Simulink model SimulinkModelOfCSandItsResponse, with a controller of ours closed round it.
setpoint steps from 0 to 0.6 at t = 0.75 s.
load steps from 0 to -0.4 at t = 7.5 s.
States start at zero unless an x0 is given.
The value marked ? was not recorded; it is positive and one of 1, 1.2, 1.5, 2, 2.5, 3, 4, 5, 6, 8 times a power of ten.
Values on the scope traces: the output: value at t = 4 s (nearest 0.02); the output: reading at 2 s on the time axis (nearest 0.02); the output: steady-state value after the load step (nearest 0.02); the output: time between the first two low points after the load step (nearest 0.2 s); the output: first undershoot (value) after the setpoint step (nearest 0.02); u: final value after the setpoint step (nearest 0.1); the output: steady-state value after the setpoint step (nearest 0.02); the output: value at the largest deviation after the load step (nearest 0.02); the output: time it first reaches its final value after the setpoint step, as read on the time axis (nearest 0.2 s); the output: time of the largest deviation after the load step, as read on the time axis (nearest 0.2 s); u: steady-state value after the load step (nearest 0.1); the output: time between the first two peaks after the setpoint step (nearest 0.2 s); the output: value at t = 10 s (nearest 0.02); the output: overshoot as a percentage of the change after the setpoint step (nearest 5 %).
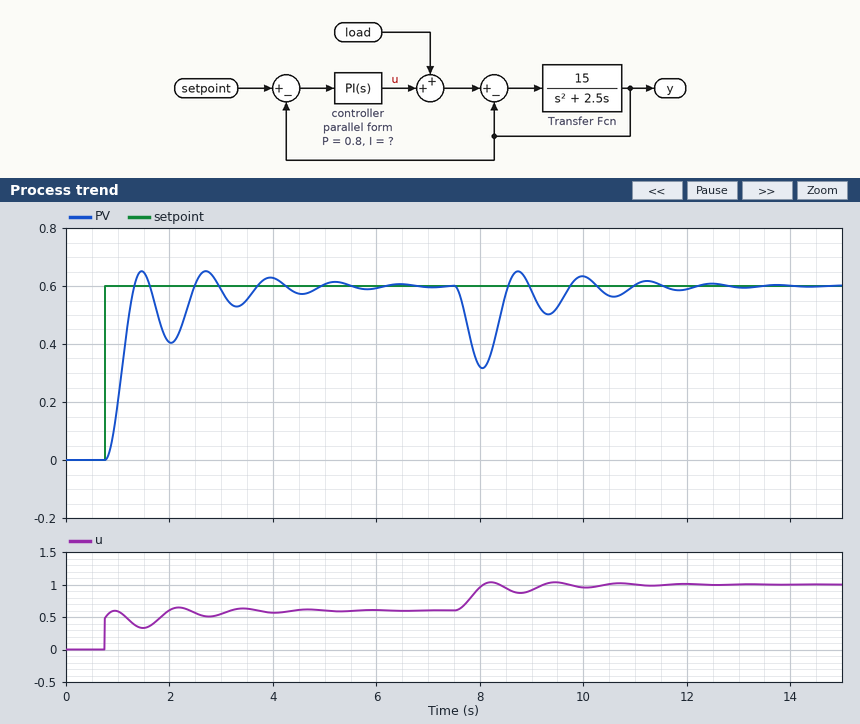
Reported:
0.62
0.40
0.60
1.2 s
0.40
0.6
0.60
0.32
1.4 s
8.0 s
1.0
1.2 s
0.64
10 %
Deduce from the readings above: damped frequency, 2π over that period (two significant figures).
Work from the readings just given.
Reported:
5.2 rad/s
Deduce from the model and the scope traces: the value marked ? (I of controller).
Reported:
2
